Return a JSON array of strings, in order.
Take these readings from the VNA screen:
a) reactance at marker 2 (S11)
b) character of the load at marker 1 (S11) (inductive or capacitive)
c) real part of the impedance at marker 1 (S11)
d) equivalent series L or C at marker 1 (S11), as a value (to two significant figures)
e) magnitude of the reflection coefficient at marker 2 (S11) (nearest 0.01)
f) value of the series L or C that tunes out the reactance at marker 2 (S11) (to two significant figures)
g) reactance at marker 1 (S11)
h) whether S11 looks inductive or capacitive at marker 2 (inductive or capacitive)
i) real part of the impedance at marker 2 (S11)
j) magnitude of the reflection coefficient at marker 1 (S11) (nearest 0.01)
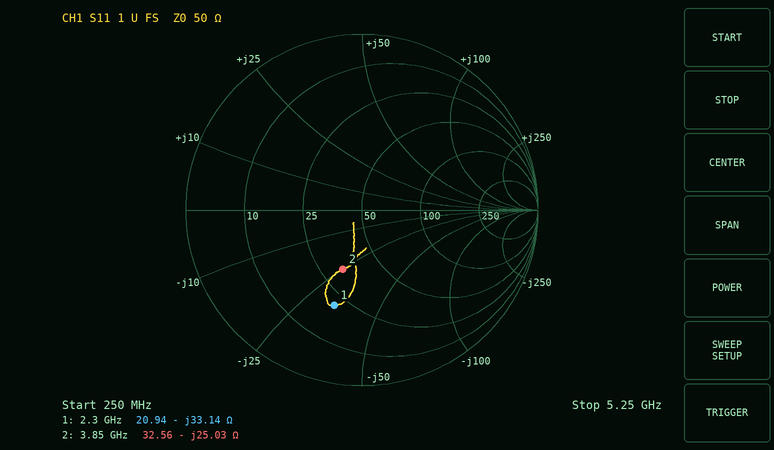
["-25.03 Ω", "capacitive", "20.94 Ω", "2.1 pF", "0.35", "1.0 nH", "-33.14 Ω", "capacitive", "32.56 Ω", "0.56"]
